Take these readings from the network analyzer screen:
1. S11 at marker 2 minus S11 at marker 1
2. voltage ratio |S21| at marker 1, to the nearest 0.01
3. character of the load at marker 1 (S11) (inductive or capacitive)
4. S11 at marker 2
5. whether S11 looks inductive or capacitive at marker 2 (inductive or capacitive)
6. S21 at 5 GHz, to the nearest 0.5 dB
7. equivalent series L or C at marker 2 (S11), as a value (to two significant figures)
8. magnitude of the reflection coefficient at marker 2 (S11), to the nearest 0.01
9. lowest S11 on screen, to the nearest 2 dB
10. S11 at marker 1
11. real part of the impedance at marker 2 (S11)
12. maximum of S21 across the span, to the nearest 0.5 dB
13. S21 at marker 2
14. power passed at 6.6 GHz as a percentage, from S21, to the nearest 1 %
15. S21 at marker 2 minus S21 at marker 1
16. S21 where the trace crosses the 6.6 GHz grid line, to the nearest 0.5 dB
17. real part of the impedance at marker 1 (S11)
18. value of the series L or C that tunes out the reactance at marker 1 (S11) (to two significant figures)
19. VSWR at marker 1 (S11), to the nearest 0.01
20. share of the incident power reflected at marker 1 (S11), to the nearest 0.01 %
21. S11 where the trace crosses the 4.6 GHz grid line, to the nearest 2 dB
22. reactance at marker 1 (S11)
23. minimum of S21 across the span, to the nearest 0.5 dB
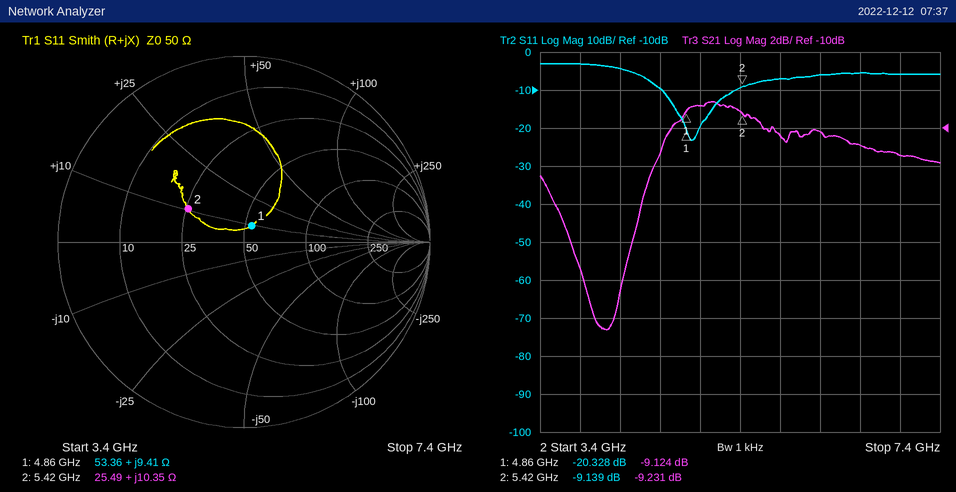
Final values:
11.189 dB
0.35
inductive
-9.139 dB
inductive
-9.0 dB
300 pH
0.35
-24 dB
-20.328 dB
25.49 Ω
-8.5 dB
-9.231 dB
8 %
-0.107 dB
-11.0 dB
53.36 Ω
3.5 pF
1.21
0.93 %
-10 dB
+9.41 Ω
-20.5 dB
